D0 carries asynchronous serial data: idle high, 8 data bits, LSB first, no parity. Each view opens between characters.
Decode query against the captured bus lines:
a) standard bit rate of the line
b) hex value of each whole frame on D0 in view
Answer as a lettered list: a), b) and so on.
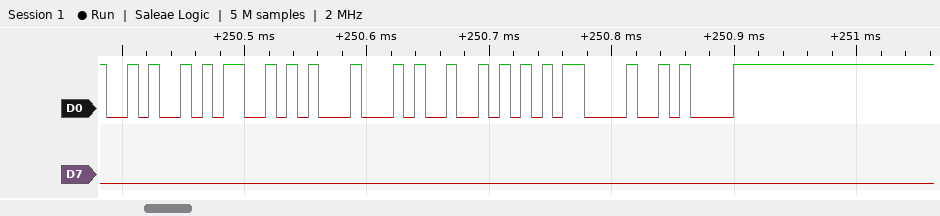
a) 115200 baud
b) 4A, 53, 44, 52, 0D, 0A
